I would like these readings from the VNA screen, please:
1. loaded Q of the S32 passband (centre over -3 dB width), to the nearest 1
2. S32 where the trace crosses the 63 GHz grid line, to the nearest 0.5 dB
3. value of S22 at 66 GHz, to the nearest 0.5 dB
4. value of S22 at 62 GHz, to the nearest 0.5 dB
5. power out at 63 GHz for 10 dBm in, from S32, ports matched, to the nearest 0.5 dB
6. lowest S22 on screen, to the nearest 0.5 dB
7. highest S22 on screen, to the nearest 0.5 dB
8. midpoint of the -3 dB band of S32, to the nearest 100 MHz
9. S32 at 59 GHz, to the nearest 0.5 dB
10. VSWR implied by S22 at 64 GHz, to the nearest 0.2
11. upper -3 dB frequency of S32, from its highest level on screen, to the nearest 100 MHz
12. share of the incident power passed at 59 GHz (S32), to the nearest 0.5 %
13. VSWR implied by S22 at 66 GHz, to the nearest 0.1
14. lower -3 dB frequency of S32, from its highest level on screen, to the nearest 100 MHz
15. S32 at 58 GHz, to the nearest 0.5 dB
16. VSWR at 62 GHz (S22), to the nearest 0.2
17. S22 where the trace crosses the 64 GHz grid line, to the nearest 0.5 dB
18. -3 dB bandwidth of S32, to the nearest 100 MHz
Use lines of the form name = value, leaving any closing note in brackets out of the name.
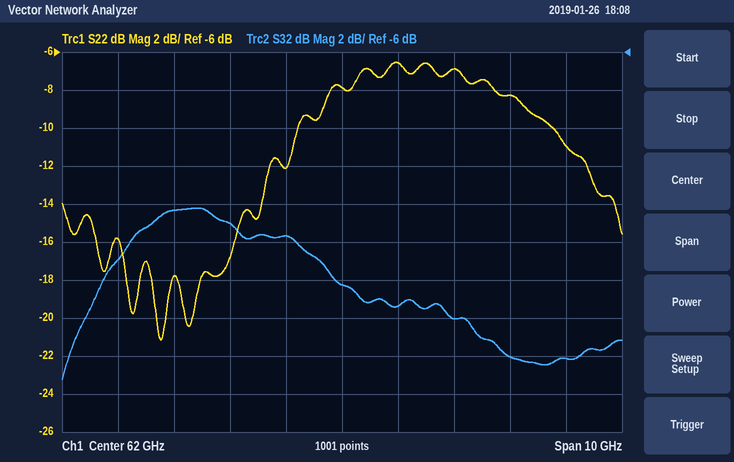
loaded Q of the S32 passband (centre over -3 dB width), to the nearest 1 = 16
S32 where the trace crosses the 63 GHz grid line, to the nearest 0.5 dB = -19.5 dB
value of S22 at 66 GHz, to the nearest 0.5 dB = -11.0 dB
value of S22 at 62 GHz, to the nearest 0.5 dB = -8.0 dB
power out at 63 GHz for 10 dBm in, from S32, ports matched, to the nearest 0.5 dB = -9.5 dBm
lowest S22 on screen, to the nearest 0.5 dB = -21.0 dB
highest S22 on screen, to the nearest 0.5 dB = -6.5 dB
midpoint of the -3 dB band of S32, to the nearest 100 MHz = 59.8 GHz
S32 at 59 GHz, to the nearest 0.5 dB = -14.5 dB
VSWR implied by S22 at 64 GHz, to the nearest 0.2 = 2.6
upper -3 dB frequency of S32, from its highest level on screen, to the nearest 100 MHz = 61.7 GHz
share of the incident power passed at 59 GHz (S32), to the nearest 0.5 % = 3.5 %
VSWR implied by S22 at 66 GHz, to the nearest 0.1 = 1.8
lower -3 dB frequency of S32, from its highest level on screen, to the nearest 100 MHz = 57.9 GHz
S32 at 58 GHz, to the nearest 0.5 dB = -17.0 dB
VSWR at 62 GHz (S22), to the nearest 0.2 = 2.4
S22 where the trace crosses the 64 GHz grid line, to the nearest 0.5 dB = -7.0 dB
-3 dB bandwidth of S32, to the nearest 100 MHz = 3.8 GHz
